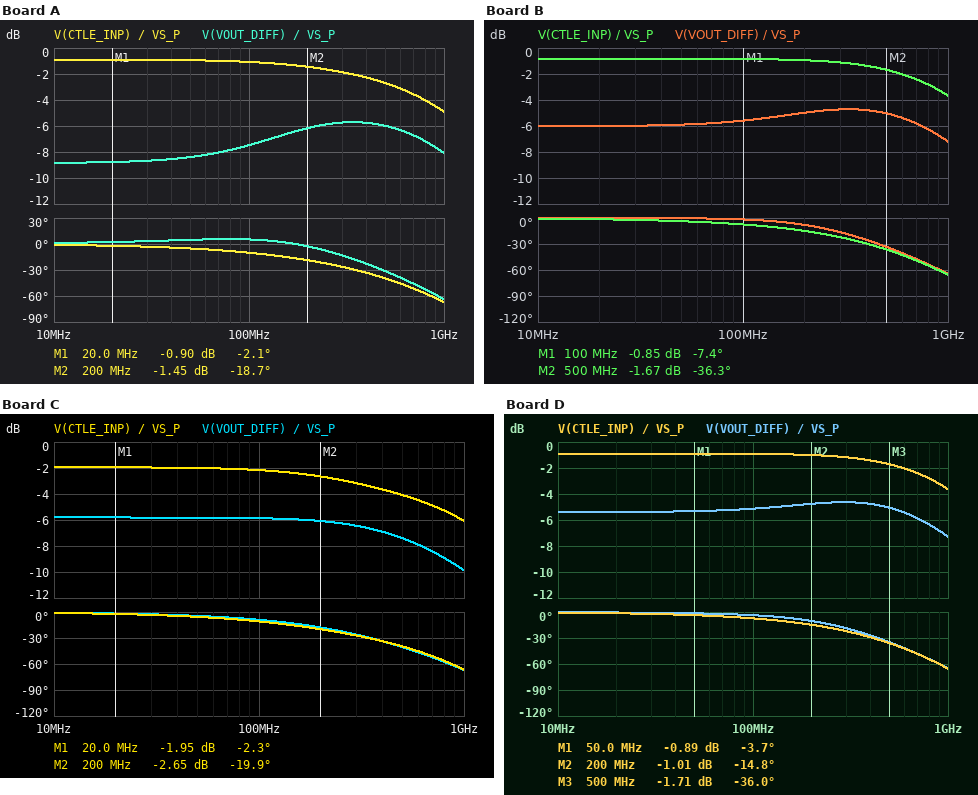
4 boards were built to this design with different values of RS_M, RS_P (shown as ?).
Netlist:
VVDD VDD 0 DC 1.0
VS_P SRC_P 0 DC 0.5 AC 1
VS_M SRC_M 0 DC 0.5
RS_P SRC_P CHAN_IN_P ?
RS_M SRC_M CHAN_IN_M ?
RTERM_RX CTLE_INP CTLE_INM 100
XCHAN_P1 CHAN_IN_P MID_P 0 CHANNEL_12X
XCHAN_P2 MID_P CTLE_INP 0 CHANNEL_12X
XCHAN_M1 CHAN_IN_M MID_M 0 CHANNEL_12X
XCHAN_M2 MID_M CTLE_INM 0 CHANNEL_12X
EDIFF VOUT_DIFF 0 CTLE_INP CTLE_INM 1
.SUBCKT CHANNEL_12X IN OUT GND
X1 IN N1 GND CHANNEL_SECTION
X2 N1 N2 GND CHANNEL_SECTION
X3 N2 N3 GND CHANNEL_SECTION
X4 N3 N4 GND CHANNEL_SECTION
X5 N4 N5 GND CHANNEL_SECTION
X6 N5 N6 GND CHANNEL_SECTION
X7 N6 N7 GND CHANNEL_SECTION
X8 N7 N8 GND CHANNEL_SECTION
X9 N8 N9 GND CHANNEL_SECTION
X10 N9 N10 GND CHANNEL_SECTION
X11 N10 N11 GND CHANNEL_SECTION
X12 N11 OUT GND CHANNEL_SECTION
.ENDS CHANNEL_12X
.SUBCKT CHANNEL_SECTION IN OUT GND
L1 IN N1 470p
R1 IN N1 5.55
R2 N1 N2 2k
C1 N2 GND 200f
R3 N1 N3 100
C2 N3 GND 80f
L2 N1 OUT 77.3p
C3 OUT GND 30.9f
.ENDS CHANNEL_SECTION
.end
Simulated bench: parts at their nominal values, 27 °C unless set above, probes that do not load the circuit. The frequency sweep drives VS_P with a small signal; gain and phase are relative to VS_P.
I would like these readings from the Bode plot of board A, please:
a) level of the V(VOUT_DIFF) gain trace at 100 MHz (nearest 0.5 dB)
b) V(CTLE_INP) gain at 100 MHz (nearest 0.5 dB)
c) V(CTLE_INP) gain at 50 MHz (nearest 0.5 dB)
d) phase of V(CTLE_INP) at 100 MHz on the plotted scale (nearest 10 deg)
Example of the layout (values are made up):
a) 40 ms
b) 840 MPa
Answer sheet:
a) -7.5 dB
b) -1.0 dB
c) -1.0 dB
d) -10 deg
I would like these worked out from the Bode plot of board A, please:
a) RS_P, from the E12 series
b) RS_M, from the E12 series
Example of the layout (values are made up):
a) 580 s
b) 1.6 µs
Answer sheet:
a) 27 Ω
b) 150 Ω
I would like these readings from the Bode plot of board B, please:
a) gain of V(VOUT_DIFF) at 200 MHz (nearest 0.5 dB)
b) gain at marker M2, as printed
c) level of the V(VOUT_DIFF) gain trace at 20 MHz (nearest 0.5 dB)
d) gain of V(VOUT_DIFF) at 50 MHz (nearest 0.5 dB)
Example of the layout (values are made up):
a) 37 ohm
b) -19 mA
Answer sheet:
a) -5.0 dB
b) -1.67 dB
c) -6.0 dB
d) -6.0 dB
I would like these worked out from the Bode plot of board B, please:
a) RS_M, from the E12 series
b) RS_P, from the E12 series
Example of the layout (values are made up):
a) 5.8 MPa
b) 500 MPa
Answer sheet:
a) 82 Ω
b) 18 Ω
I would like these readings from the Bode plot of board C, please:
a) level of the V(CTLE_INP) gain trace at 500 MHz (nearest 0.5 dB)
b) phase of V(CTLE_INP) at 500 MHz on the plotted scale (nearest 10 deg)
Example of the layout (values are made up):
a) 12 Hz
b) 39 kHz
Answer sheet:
a) -4.0 dB
b) -40 deg
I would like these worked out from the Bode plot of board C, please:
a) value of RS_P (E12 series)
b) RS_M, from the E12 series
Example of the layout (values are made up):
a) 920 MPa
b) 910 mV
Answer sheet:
a) 39 Ω
b) 56 Ω
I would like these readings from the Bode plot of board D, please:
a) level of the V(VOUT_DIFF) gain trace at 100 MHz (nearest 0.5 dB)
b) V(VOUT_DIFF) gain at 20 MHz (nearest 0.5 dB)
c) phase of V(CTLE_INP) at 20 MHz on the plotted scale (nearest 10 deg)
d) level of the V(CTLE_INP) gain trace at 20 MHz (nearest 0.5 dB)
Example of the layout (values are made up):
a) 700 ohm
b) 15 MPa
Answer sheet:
a) -5.0 dB
b) -5.5 dB
c) 0 deg
d) -1.0 dB
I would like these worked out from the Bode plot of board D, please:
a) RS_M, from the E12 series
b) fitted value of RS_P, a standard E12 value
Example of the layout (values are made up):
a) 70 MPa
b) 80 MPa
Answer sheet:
a) 68 Ω
b) 18 Ω
